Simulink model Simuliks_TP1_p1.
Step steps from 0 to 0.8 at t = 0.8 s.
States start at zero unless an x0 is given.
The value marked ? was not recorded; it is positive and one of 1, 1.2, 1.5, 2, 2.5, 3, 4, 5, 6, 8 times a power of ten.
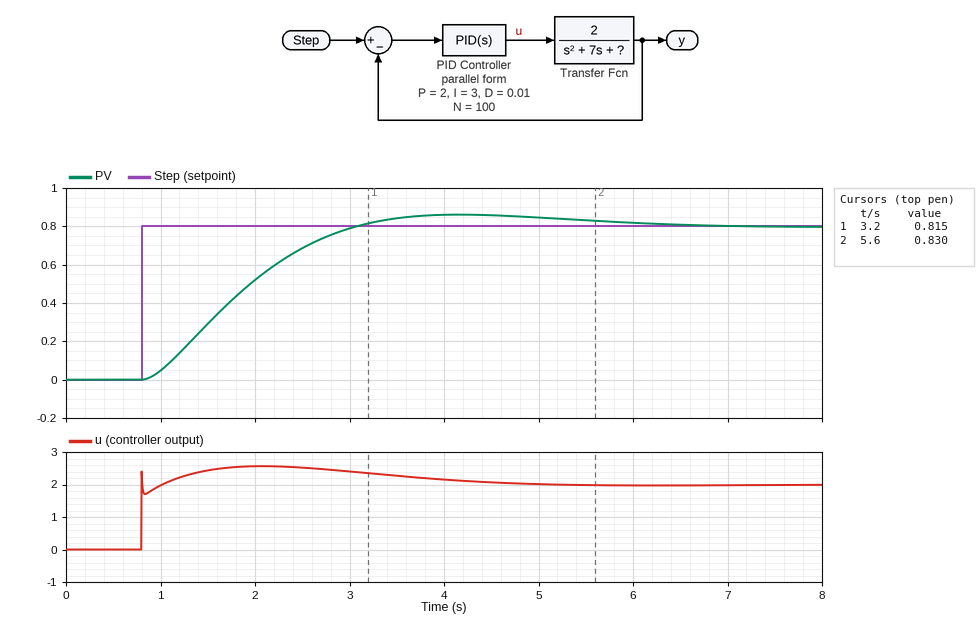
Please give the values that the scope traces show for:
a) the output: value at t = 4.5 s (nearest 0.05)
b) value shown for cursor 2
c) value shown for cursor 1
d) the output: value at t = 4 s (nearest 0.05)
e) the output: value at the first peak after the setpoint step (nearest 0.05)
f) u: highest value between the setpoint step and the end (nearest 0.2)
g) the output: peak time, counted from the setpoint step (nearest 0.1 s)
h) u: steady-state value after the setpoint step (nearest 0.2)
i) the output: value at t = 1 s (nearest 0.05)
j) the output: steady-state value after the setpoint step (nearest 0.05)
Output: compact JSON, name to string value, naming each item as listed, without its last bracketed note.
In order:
{"the output: value at t = 4.5 s": "0.85", "value shown for cursor 2": "0.830", "value shown for cursor 1": "0.815", "the output: value at t = 4 s": "0.85", "the output: value at the first peak after the setpoint step": "0.85", "u: highest value between the setpoint step and the end": "2.6", "the output: peak time, counted from the setpoint step": "3.4 s", "u: steady-state value after the setpoint step": "2.0", "the output: value at t = 1 s": "0.05", "the output: steady-state value after the setpoint step": "0.80"}
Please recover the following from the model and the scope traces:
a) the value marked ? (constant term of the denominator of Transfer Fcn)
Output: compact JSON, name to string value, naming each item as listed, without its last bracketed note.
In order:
{"the value marked ?": "5"}
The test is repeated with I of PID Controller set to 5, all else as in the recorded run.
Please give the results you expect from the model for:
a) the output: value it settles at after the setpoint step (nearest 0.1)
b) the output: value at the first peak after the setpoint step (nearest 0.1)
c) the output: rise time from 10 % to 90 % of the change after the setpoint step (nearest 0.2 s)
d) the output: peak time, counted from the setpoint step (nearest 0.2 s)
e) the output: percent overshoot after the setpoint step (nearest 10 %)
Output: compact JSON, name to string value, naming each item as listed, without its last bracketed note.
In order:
{"the output: value it settles at after the setpoint step": "0.8", "the output: value at the first peak after the setpoint step": "1.0", "the output: rise time from 10 % to 90 % of the change after the setpoint step": "1.0 s", "the output: peak time, counted from the setpoint step": "2.4 s", "the output: percent overshoot after the setpoint step": "20 %"}
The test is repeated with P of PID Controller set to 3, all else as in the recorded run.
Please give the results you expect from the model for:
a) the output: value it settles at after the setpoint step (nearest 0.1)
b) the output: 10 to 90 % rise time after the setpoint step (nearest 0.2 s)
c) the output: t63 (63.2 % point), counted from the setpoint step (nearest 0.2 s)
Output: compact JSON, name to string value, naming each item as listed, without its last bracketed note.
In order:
{"the output: value it settles at after the setpoint step": "0.8", "the output: 10 to 90 % rise time after the setpoint step": "1.6 s", "the output: t63 (63.2 % point), counted from the setpoint step": "1.0 s"}
